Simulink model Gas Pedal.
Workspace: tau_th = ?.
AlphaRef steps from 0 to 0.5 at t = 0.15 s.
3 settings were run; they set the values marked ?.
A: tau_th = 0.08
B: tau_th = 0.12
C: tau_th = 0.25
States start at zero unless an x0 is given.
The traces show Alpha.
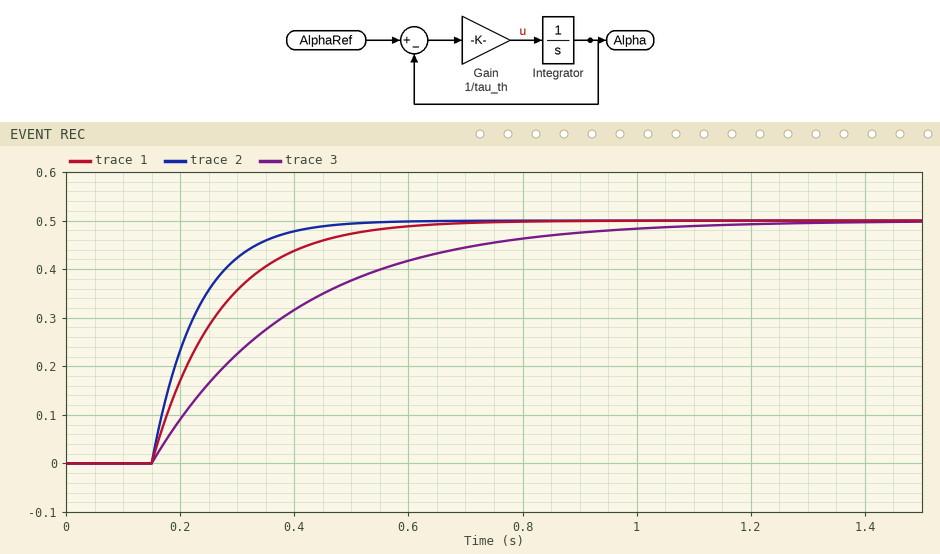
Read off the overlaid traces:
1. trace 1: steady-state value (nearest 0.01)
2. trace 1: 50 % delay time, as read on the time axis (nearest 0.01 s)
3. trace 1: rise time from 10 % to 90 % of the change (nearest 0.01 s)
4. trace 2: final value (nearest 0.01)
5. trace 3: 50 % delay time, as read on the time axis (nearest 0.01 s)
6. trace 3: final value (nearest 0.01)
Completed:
0.50
0.23 s
0.26 s
0.50
0.32 s
0.50
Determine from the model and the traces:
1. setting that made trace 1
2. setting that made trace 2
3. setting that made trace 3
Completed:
B
A
C
